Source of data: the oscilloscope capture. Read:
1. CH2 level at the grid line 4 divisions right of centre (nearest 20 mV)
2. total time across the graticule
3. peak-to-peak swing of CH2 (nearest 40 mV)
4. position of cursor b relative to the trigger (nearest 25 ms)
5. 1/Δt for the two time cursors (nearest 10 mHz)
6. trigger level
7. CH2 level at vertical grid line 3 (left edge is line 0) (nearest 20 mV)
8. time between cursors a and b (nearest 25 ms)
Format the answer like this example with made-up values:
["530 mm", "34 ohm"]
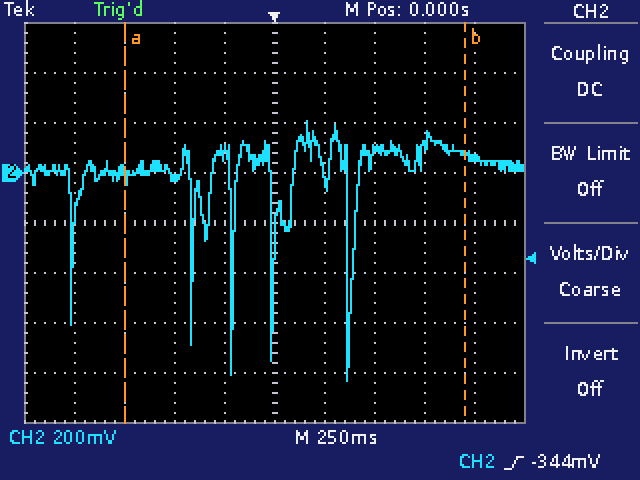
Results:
["60 mV", "2.5 s", "1.04 V", "+950 ms", "590 mHz", "-344 mV", "-20 mV", "1.700 s"]
